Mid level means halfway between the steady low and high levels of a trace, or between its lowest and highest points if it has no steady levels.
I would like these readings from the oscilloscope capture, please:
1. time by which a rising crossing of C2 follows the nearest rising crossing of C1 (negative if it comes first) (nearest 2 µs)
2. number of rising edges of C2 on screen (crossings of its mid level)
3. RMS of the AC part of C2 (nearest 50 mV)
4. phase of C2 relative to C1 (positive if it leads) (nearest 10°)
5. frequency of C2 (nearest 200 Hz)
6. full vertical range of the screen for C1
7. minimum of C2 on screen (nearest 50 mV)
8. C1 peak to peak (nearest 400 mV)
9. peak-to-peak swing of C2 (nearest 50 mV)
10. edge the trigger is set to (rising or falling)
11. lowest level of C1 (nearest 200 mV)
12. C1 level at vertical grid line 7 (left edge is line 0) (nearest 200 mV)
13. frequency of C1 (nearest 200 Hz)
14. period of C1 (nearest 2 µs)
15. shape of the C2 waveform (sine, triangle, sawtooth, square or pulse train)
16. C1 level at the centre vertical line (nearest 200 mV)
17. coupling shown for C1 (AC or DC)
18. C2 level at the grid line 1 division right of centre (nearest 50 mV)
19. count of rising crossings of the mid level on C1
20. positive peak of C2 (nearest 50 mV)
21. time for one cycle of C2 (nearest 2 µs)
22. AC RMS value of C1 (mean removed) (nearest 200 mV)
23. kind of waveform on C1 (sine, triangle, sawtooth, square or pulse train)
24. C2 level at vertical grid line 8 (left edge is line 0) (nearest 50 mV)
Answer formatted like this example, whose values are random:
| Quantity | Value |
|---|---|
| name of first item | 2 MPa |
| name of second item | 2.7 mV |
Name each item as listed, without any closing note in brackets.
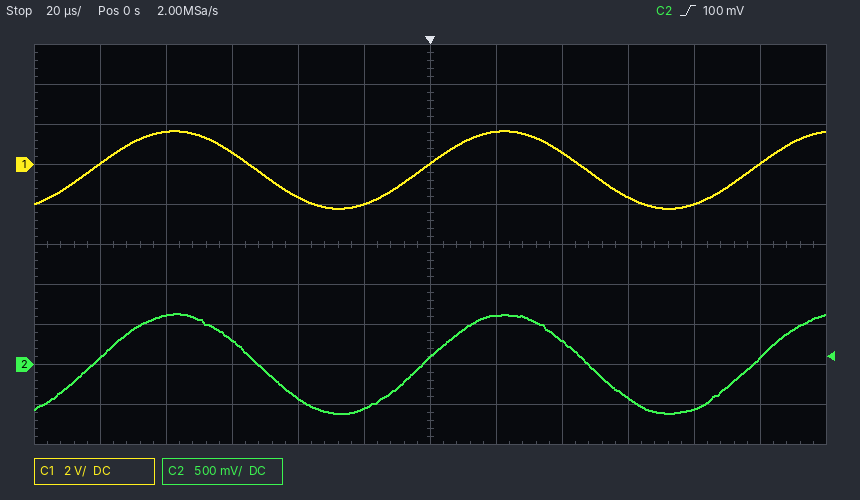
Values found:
| Quantity | Value |
|---|---|
| time by which a rising crossing of C2 follows the nearest rising crossing of C1 (negative if it comes first) | 0 µs |
| number of rising edges of C2 on screen | 3 |
| RMS of the AC part of C2 | 450 mV |
| phase of C2 relative to C1 (positive if it leads) | 0° |
| frequency of C2 | 10.0 kHz |
| full vertical range of the screen for C1 | 20 V |
| minimum of C2 on screen | -600 mV |
| C1 peak to peak | 4.0 V |
| peak-to-peak swing of C2 | 1.25 V |
| edge the trigger is set to | rising |
| lowest level of C1 | -2.2 V |
| C1 level at vertical grid line 7 (left edge is line 0) | 1.6 V |
| frequency of C1 | 10.0 kHz |
| period of C1 | 100 µs |
| shape of the C2 waveform | sine |
| C1 level at the centre vertical line | 0.0 V |
| coupling shown for C1 | DC |
| C2 level at the grid line 1 division right of centre | 600 mV |
| count of rising crossings of the mid level on C1 | 3 |
| positive peak of C2 | 650 mV |
| time for one cycle of C2 | 100 µs |
| AC RMS value of C1 (mean removed) | 1.4 V |
| kind of waveform on C1 | sine |
| C2 level at vertical grid line 8 (left edge is line 0) | 300 mV |
